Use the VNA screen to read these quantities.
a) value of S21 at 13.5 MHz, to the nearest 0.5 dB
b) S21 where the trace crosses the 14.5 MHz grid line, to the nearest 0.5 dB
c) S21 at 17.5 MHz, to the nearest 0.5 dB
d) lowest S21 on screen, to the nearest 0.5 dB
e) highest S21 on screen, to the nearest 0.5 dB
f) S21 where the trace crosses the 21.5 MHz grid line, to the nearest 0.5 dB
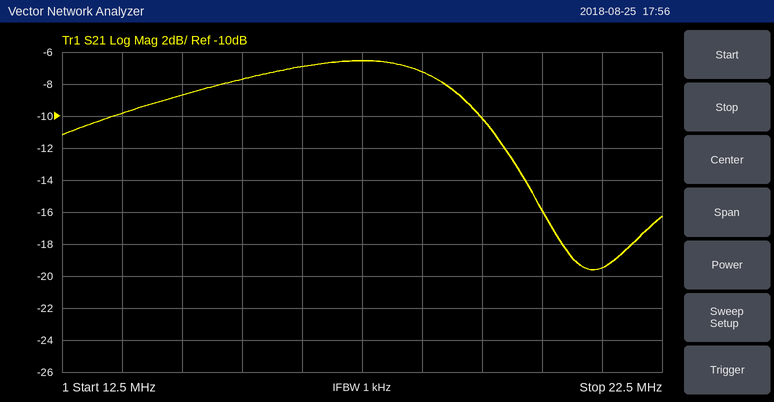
-10.0 dB
-8.5 dB
-6.5 dB
-19.5 dB
-6.5 dB
-19.5 dB
